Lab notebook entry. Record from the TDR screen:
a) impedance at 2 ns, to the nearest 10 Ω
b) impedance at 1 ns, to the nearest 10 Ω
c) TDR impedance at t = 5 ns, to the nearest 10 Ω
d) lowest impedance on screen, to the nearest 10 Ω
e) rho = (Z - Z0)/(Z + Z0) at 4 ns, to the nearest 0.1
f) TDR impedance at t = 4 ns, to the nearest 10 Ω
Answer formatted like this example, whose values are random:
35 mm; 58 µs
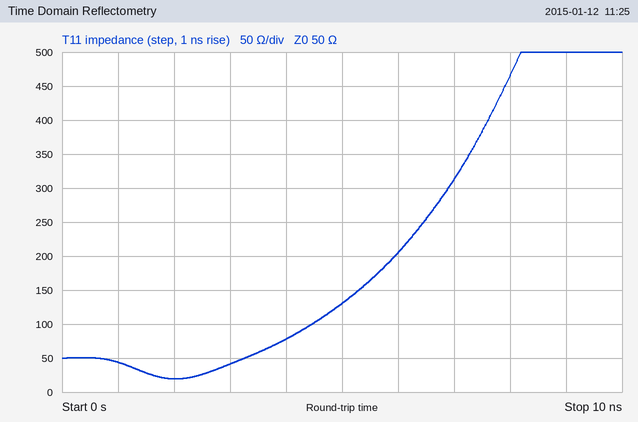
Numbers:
20 Ω; 40 Ω; 130 Ω; 20 Ω; +0.2; 80 Ω
